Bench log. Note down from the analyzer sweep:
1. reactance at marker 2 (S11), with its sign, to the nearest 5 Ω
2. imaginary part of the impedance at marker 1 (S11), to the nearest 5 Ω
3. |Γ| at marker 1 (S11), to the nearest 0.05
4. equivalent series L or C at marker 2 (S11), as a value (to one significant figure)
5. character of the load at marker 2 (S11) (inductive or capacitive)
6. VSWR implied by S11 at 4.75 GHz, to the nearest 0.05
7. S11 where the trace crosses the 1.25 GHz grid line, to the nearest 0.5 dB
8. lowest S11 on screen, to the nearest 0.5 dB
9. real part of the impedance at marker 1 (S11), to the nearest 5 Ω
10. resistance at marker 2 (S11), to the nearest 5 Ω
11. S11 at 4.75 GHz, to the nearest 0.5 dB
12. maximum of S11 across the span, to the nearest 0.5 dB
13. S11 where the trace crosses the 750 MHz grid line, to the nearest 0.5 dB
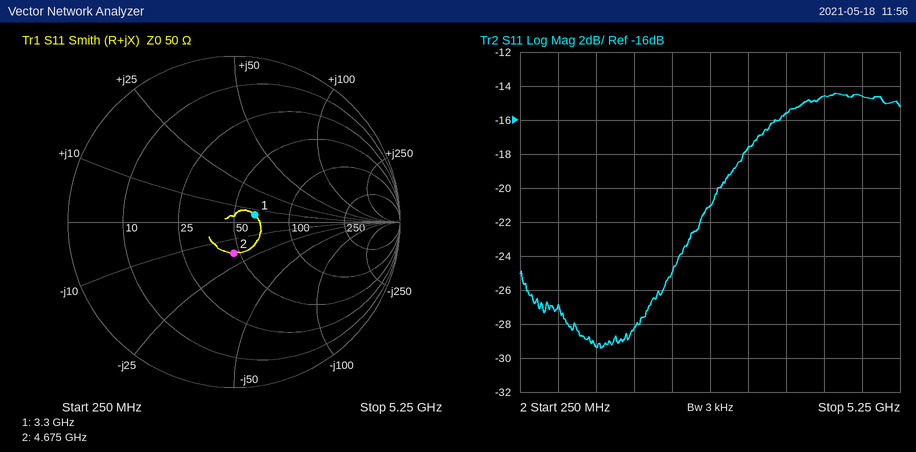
-20 Ω
+5 Ω
0.15
2 pF
capacitive
1.45
-29.5 dB
-29.5 dB
65 Ω
45 Ω
-14.5 dB
-14.5 dB
-27.0 dB
